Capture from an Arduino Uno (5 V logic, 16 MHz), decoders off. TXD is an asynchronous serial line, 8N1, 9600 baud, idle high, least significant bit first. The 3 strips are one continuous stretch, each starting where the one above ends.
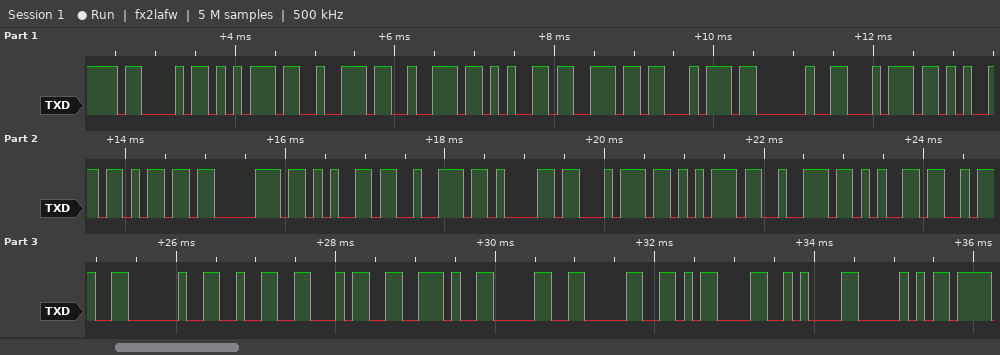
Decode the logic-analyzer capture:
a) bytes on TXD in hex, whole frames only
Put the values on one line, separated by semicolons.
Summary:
43 75 72 72 65 6E 74 20 74 65 6D 70 65 72 61 74 75 72 65 3A 20 32 34 2E 30 30 0D 0A 50
